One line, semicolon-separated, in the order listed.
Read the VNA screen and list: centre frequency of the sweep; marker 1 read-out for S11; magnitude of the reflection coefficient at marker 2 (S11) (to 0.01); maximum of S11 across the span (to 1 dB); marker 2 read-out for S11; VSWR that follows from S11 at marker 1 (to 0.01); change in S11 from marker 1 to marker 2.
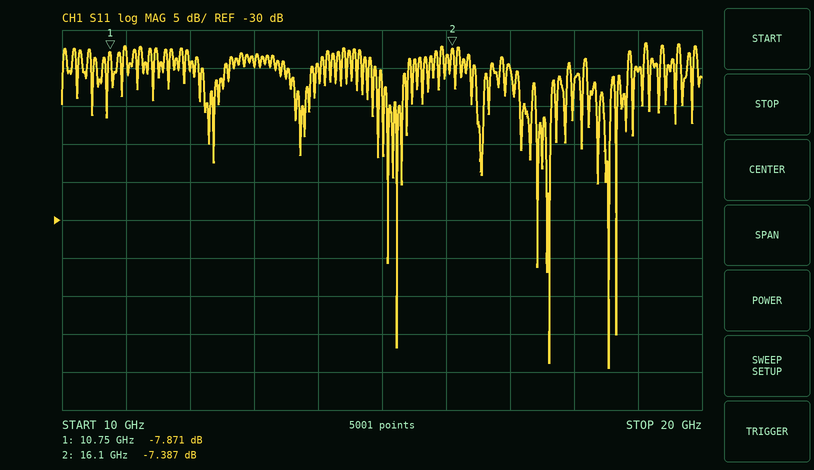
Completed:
15 GHz; -7.871 dB; 0.43; -7 dB; -7.387 dB; 2.36; 0.484 dB
